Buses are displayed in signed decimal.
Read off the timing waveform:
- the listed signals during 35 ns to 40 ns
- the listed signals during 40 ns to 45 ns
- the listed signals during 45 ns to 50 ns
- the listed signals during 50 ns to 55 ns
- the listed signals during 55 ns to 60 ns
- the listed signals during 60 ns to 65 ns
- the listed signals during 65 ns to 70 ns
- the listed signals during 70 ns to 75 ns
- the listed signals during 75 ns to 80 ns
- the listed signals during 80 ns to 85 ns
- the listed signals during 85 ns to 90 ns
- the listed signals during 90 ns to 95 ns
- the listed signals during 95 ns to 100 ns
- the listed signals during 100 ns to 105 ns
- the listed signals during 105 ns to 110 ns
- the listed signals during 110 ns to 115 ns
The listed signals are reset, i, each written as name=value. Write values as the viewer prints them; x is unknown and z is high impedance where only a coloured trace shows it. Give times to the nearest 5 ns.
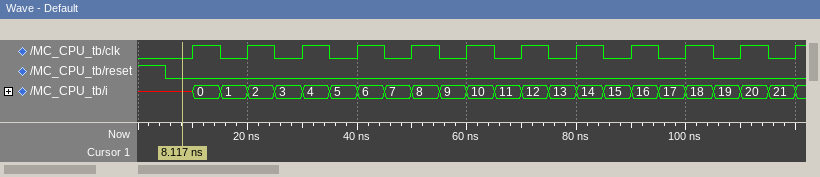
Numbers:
reset=0, i=5
reset=0, i=6
reset=0, i=7
reset=0, i=8
reset=0, i=9
reset=0, i=10
reset=0, i=11
reset=0, i=12
reset=0, i=13
reset=0, i=14
reset=0, i=15
reset=0, i=16
reset=0, i=17
reset=0, i=18
reset=0, i=19
reset=0, i=20
